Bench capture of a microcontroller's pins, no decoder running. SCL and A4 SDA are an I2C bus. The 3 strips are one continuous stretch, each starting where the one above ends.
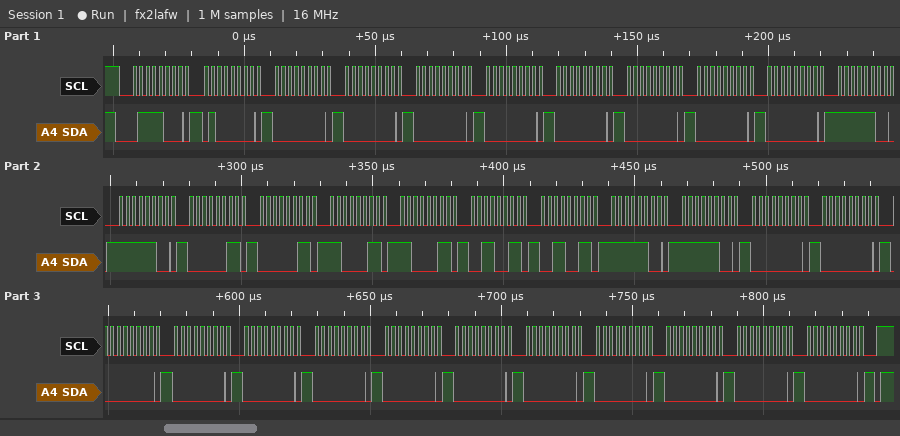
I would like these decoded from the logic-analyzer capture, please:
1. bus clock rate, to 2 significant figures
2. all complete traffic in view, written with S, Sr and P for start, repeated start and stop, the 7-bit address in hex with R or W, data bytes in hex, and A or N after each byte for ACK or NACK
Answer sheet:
400 kHz
S 3CW A 40 A 00 A 00 A 00 A 00 A 00 A 00 A 00 A 00 A FC A FC A 03 A 03 A C3 A C3 A 33 A 33 A FC A FC A 00 A 00 A 00 A 00 A 00 A 00 A 00 A 00 A 00 A 00 A 00 A 00 A 00 A P
